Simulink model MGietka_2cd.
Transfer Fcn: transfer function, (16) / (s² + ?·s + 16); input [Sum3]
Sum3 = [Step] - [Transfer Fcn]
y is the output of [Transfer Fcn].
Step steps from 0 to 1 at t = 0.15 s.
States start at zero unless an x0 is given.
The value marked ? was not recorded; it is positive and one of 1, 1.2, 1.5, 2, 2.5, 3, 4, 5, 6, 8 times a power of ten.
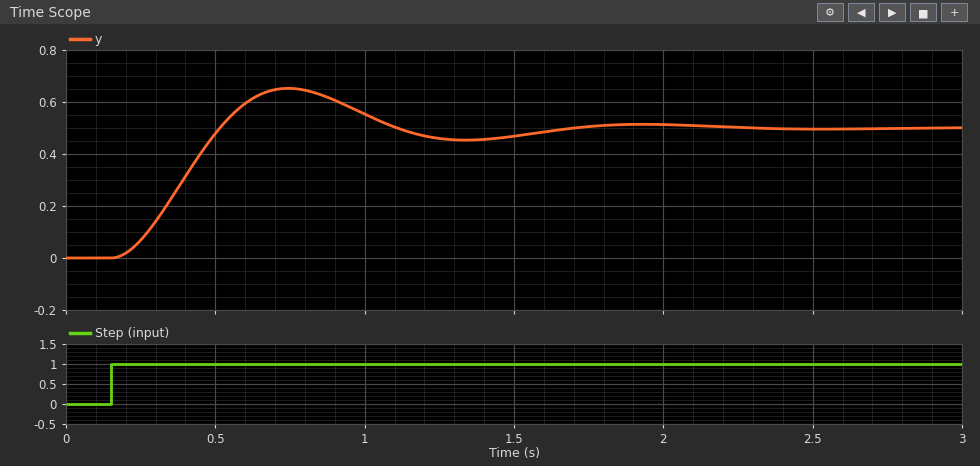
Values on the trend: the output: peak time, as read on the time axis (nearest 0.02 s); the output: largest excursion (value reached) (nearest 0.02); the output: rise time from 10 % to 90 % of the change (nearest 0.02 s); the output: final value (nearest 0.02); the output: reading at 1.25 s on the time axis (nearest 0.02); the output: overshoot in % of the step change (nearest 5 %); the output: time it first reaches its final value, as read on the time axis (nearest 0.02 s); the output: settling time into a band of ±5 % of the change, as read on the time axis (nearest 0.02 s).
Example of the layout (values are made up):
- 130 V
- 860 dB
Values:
- 0.74 s
- 0.66
- 0.24 s
- 0.50
- 0.46
- 30 %
- 0.52 s
- 1.54 s
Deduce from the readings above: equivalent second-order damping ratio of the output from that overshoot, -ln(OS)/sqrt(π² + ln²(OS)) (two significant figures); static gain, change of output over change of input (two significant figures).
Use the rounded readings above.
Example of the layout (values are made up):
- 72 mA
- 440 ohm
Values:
- 0.36
- 0.50
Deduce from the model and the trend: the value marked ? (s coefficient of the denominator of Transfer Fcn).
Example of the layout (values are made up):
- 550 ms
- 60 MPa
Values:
- 4
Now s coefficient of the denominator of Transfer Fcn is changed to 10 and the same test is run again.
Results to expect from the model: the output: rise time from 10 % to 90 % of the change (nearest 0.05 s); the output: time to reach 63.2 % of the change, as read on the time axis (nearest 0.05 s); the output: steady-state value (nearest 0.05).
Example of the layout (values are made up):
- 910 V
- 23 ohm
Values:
- 0.50 s
- 0.50 s
- 0.50
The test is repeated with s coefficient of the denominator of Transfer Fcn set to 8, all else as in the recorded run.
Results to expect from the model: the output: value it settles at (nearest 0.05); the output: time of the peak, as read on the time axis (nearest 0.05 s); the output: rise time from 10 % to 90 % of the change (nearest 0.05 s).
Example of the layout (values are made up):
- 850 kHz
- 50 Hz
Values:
- 0.50
- 0.95 s
- 0.40 s
